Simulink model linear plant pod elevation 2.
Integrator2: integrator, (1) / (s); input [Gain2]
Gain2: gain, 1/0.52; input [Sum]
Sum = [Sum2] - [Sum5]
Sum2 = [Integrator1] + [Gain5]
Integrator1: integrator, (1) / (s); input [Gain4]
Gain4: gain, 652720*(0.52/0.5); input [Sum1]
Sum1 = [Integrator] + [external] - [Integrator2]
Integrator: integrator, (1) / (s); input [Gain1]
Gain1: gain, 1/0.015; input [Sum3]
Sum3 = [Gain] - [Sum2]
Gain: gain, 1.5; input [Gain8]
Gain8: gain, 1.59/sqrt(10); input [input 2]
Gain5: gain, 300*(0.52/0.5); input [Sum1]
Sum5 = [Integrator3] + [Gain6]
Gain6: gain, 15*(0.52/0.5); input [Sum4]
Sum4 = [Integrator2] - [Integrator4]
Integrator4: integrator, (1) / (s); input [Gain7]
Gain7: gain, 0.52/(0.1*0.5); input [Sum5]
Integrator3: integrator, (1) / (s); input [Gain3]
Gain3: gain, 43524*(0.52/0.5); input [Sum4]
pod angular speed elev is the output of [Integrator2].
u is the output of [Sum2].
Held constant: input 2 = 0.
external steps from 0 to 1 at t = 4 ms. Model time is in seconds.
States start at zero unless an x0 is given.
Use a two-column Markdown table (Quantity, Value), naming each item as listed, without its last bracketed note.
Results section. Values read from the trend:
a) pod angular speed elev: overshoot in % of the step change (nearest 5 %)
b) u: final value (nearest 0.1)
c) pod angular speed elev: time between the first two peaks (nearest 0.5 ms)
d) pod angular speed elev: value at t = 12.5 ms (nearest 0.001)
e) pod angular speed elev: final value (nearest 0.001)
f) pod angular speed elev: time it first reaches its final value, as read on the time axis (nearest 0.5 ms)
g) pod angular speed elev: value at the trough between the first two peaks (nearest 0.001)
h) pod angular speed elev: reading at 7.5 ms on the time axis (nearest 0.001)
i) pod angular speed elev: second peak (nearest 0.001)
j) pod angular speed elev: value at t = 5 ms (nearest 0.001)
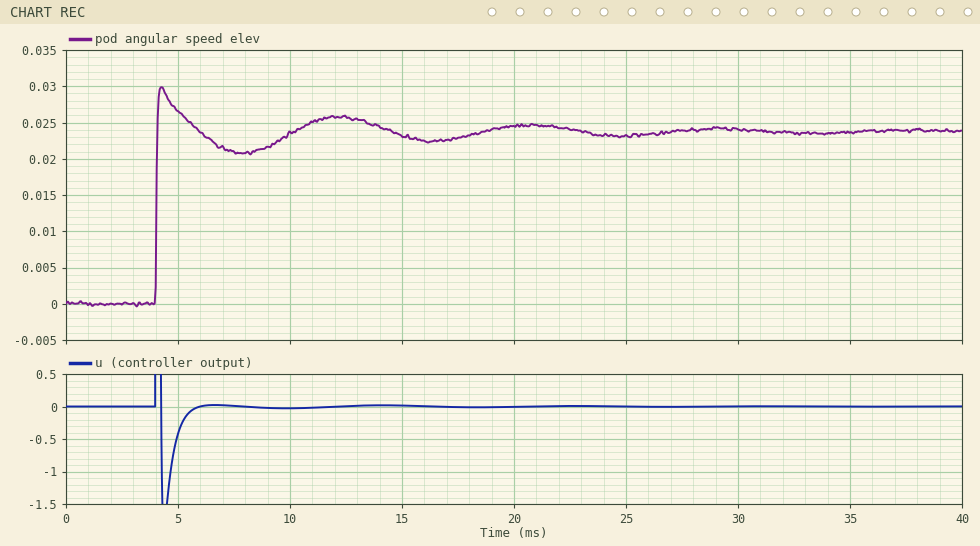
| Quantity | Value |
|---|---|
| pod angular speed elev: overshoot in % of the step change | 25 % |
| u: final value | 0.0 |
| pod angular speed elev: time between the first two peaks | 8.0 ms |
| pod angular speed elev: value at t = 12.5 ms | 0.026 |
| pod angular speed elev: final value | 0.024 |
| pod angular speed elev: time it first reaches its final value, as read on the time axis | 4.0 ms |
| pod angular speed elev: value at the trough between the first two peaks | 0.021 |
| pod angular speed elev: reading at 7.5 ms on the time axis | 0.021 |
| pod angular speed elev: second peak | 0.026 |
| pod angular speed elev: value at t = 5 ms | 0.027 |
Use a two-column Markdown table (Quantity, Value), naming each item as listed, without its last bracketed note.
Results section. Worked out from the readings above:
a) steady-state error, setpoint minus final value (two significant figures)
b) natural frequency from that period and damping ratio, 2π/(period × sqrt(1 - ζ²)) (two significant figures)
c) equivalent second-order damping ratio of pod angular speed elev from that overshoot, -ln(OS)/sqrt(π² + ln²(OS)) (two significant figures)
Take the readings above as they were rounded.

| Quantity | Value |
|---|---|
| steady-state error, setpoint minus final value | 0.98 |
| natural frequency from that period and damping ratio, 2π/(period × sqrt(1 - ζ²)) | 0.86 rad/ms |
| equivalent second-order damping ratio of pod angular speed elev from that overshoot, -ln(OS)/sqrt(π² + ln²(OS)) | 0.40 |
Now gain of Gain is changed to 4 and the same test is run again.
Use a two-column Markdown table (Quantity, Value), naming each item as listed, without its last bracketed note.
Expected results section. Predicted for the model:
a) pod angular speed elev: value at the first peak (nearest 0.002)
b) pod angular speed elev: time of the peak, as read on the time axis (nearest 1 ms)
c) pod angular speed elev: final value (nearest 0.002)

| Quantity | Value |
|---|---|
| pod angular speed elev: value at the first peak | 0.030 |
| pod angular speed elev: time of the peak, as read on the time axis | 4 ms |
| pod angular speed elev: final value | 0.024 |
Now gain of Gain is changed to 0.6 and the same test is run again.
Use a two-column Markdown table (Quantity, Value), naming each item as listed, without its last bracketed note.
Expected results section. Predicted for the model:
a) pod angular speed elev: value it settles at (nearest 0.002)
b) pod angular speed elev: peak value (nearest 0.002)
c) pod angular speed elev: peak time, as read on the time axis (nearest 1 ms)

| Quantity | Value |
|---|---|
| pod angular speed elev: value it settles at | 0.024 |
| pod angular speed elev: peak value | 0.030 |
| pod angular speed elev: peak time, as read on the time axis | 4 ms |
